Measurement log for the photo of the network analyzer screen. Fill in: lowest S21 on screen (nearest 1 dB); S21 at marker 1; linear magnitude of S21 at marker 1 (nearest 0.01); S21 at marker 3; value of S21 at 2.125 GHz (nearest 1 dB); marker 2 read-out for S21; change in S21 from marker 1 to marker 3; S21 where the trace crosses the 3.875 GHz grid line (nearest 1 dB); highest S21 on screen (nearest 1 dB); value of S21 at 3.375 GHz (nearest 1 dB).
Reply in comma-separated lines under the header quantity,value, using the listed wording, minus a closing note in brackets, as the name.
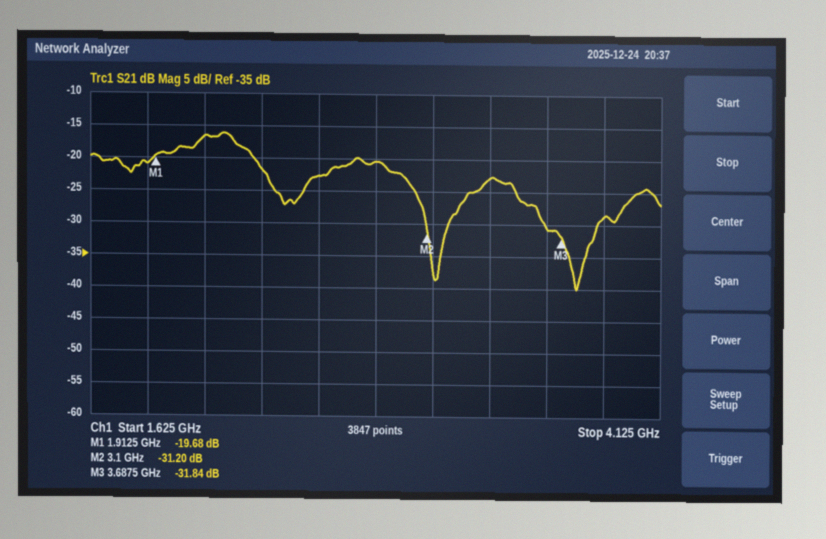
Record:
quantity,value
lowest S21 on screen,-40 dB
S21 at marker 1,-19.68 dB
linear magnitude of S21 at marker 1,0.10
S21 at marker 3,-31.84 dB
value of S21 at 2.125 GHz,-17 dB
marker 2 read-out for S21,-31.20 dB
change in S21 from marker 1 to marker 3,-12.16 dB
S21 where the trace crosses the 3.875 GHz grid line,-29 dB
highest S21 on screen,-16 dB
value of S21 at 3.375 GHz,-23 dB
